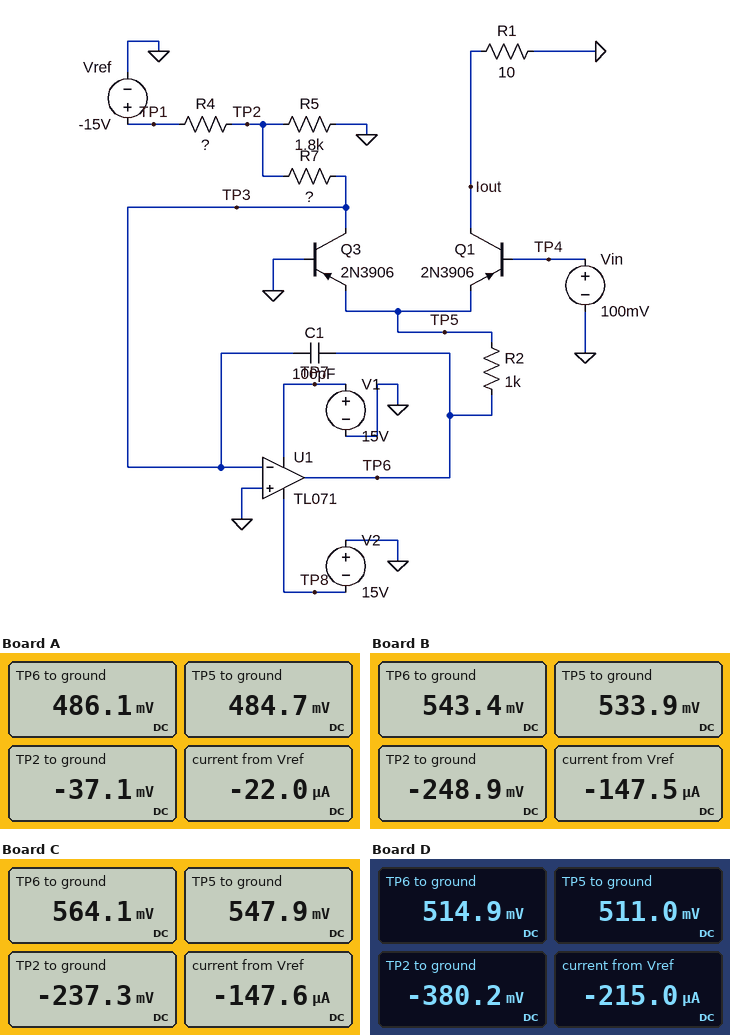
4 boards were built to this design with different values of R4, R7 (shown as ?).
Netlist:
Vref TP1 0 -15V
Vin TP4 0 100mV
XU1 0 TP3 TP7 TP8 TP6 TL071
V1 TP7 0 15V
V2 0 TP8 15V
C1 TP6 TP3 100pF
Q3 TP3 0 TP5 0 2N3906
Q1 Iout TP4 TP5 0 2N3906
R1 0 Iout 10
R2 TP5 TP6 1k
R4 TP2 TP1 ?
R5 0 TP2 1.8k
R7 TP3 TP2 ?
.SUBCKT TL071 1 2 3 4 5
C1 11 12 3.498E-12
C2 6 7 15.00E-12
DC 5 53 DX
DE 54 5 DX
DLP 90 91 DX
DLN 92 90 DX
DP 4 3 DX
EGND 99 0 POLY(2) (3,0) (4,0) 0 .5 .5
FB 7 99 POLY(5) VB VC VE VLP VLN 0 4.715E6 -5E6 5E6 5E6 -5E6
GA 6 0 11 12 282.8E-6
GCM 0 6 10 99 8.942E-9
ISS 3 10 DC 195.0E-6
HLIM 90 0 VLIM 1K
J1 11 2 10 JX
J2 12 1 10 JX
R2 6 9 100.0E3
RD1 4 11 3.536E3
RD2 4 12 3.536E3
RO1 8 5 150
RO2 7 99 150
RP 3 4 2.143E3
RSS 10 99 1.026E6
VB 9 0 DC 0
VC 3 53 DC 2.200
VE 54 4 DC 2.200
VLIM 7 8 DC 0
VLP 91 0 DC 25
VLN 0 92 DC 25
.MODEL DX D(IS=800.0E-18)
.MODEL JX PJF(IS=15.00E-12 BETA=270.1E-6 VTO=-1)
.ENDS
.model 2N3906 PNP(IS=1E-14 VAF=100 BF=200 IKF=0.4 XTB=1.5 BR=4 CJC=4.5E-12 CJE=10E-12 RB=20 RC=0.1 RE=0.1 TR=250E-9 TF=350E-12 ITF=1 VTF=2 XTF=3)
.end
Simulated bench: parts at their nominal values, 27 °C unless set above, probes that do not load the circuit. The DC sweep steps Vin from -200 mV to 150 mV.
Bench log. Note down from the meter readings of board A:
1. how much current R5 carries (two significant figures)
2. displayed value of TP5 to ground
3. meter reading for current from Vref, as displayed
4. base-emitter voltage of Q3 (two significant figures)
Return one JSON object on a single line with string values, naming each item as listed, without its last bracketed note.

{"how much current R5 carries": "21 µA", "displayed value of TP5 to ground": "484.7 mV", "meter reading for current from Vref, as displayed": "-22.0 µA", "base-emitter voltage of Q3": "-480 mV"}
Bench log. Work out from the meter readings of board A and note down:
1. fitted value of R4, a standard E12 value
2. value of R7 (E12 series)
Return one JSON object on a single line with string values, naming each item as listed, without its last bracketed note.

{"fitted value of R4, a standard E12 value": "680 kΩ", "value of R7": "27 kΩ"}
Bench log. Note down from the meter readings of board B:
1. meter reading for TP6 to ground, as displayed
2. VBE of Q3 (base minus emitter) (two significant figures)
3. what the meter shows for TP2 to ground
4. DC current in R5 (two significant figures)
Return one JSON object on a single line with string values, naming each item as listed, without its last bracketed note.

{"meter reading for TP6 to ground, as displayed": "543.4 mV", "VBE of Q3 (base minus emitter)": "-530 mV", "what the meter shows for TP2 to ground": "-248.9 mV", "DC current in R5": "140 µA"}
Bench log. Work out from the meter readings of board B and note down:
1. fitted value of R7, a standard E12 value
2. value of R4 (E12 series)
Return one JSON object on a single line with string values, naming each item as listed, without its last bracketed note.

{"fitted value of R7, a standard E12 value": "27 kΩ", "value of R4": "100 kΩ"}
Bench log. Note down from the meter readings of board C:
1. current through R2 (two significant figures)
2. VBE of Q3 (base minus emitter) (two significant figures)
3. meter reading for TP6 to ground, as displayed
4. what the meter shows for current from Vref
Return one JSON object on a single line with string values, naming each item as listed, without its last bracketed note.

{"current through R2": "16 µA", "VBE of Q3 (base minus emitter)": "-550 mV", "meter reading for TP6 to ground, as displayed": "564.1 mV", "what the meter shows for current from Vref": "-147.6 µA"}
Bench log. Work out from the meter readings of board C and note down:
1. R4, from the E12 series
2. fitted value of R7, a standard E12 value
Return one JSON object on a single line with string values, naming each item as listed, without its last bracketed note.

{"R4, from the E12 series": "100 kΩ", "fitted value of R7, a standard E12 value": "15 kΩ"}
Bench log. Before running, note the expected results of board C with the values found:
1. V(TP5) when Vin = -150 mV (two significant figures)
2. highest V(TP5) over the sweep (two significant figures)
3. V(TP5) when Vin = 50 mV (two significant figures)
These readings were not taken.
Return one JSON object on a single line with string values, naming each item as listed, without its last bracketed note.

{"V(TP5) when Vin = -150 mV": "550 mV", "highest V(TP5) over the sweep": "550 mV", "V(TP5) when Vin = 50 mV": "550 mV"}
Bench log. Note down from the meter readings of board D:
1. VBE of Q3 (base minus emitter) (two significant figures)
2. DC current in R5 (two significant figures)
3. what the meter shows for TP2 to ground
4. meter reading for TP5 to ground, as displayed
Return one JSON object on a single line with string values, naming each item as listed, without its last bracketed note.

{"VBE of Q3 (base minus emitter)": "-510 mV", "DC current in R5": "210 µA", "what the meter shows for TP2 to ground": "-380.2 mV", "meter reading for TP5 to ground, as displayed": "511.0 mV"}
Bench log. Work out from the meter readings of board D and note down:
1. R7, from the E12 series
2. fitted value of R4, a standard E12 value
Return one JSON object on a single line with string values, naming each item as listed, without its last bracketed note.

{"R7, from the E12 series": "100 kΩ", "fitted value of R4, a standard E12 value": "68 kΩ"}
